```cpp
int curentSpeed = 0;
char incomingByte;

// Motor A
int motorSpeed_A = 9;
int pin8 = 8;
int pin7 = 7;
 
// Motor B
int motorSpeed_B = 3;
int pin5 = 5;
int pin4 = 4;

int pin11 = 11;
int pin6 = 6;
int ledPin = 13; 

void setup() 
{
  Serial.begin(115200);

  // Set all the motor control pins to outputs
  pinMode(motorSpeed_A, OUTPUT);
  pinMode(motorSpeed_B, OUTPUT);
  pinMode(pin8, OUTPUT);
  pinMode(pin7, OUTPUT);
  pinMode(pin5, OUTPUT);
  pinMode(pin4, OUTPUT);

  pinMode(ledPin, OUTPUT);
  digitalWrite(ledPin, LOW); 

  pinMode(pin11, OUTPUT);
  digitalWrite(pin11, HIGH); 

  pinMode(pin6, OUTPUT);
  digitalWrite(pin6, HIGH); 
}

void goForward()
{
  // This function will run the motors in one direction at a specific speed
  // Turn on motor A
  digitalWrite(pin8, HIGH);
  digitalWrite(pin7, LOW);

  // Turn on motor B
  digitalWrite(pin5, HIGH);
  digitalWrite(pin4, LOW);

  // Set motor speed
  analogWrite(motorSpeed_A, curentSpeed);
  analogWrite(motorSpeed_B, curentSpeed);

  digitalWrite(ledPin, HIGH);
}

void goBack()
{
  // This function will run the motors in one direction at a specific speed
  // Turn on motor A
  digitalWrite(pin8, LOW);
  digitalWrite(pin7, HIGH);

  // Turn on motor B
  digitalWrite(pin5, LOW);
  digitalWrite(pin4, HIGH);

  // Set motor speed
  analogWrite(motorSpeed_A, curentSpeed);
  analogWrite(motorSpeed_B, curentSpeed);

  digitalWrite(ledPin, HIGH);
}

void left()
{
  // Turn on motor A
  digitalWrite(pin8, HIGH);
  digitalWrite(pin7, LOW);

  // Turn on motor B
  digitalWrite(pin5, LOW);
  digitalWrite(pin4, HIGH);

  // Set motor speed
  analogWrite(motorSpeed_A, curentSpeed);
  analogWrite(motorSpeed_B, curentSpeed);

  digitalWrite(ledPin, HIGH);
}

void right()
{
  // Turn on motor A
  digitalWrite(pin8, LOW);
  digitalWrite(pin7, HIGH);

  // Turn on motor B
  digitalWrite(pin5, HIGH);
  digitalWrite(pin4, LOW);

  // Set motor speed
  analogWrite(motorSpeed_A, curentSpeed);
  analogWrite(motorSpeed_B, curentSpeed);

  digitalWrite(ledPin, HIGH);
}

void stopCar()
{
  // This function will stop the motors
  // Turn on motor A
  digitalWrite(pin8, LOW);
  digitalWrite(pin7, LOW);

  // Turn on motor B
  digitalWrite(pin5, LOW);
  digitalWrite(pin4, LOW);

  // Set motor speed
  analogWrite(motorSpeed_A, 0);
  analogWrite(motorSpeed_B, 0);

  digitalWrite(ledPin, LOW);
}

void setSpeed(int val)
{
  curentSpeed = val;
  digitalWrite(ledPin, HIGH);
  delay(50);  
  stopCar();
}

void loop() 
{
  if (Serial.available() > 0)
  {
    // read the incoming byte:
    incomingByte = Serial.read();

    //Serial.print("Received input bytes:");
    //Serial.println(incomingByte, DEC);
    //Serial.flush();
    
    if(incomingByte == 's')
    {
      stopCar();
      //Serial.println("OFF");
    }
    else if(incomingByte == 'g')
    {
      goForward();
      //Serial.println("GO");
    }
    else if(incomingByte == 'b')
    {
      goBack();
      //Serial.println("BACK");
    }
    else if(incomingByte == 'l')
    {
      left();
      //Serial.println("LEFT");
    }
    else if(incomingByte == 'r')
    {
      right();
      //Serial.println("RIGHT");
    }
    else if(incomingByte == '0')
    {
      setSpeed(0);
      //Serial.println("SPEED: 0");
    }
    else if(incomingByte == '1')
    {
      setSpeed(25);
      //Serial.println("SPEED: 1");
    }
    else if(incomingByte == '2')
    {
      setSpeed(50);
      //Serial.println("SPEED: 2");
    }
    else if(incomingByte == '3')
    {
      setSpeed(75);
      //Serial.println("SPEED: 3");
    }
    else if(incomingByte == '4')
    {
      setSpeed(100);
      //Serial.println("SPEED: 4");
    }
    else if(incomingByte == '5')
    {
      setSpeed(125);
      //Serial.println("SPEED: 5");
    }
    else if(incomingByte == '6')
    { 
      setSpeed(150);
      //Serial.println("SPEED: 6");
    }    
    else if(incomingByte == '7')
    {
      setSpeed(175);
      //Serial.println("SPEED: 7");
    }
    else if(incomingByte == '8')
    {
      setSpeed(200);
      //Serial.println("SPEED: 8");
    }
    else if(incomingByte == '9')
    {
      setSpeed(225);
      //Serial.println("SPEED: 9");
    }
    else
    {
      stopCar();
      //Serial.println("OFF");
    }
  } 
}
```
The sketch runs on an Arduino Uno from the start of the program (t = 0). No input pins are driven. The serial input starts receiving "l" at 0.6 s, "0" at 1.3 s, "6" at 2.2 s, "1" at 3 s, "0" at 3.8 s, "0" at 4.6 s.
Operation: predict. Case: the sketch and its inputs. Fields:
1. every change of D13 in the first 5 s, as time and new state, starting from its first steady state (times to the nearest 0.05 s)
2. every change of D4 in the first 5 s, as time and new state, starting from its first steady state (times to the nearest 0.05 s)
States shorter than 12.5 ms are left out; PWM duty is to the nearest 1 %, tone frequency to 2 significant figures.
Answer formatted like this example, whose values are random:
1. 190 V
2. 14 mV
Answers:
1. 0 s low; 0.6 s high; 1.35 s low; 2.2 s high; 2.25 s low; 3 s high; 3.05 s low; 3.8 s high; 3.85 s low; 4.6 s high; 4.65 s low
2. 0 s low; 0.6 s high; 1.35 s low
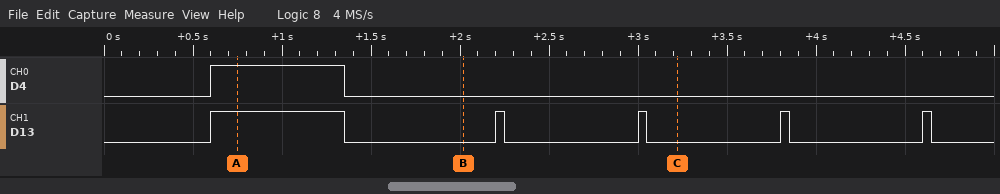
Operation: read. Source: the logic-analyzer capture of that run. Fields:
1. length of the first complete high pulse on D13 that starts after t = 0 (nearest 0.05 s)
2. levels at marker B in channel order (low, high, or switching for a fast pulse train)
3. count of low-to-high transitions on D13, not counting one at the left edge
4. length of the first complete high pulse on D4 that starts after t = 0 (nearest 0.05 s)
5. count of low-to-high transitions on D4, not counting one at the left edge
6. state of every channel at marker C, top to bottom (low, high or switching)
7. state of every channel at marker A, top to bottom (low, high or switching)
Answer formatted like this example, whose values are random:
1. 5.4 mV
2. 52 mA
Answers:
1. 0.75 s
2. D4 low, D13 low
3. 5
4. 0.75 s
5. 1
6. D4 low, D13 low
7. D4 high, D13 high
